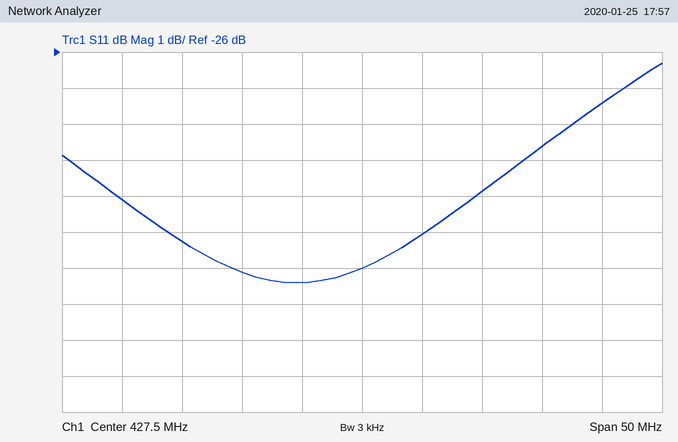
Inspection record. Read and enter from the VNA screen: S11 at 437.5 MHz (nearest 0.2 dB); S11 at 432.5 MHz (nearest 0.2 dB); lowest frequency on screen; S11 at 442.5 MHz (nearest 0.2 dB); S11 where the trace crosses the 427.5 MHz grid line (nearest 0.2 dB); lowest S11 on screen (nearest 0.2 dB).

-29.8 dB
-31.0 dB
402.5 MHz
-28.6 dB
-32.0 dB
-32.4 dB
